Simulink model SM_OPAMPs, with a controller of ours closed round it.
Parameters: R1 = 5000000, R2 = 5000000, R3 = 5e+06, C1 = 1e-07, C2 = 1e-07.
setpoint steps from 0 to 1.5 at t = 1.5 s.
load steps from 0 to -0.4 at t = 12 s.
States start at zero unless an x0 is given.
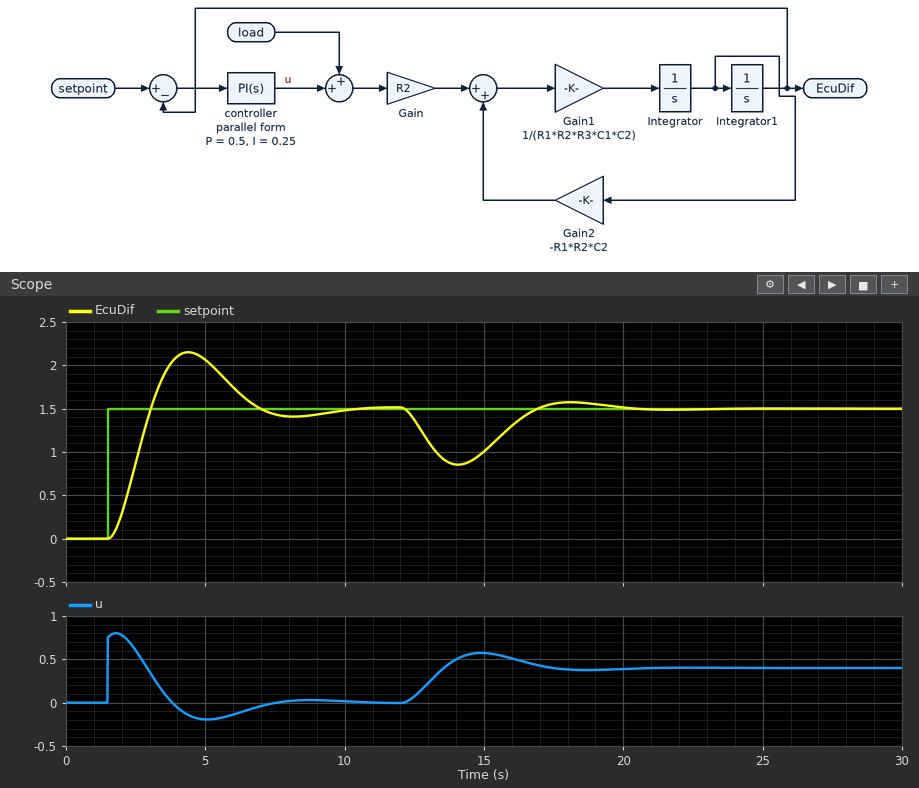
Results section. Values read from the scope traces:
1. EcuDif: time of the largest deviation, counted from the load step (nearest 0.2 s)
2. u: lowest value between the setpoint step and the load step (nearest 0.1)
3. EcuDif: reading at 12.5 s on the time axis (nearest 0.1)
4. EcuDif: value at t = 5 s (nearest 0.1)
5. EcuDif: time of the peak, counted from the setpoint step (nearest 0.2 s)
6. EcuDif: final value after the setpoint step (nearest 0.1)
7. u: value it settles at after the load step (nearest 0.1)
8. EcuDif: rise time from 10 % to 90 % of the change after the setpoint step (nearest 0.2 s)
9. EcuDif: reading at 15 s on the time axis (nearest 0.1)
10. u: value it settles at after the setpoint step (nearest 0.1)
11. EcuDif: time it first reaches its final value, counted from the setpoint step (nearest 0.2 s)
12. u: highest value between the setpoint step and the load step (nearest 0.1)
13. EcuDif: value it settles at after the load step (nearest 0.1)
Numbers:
2.0 s
-0.2
1.4
2.1
2.8 s
1.5
0.4
1.0 s
1.0
0.0
1.6 s
0.8
1.5
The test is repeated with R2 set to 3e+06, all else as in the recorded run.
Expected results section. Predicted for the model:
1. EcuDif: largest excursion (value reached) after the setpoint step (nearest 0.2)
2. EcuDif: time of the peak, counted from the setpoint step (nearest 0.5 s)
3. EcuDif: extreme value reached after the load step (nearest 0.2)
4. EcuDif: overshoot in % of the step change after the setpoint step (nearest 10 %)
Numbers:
2.2
3.0 s
0.8
40 %
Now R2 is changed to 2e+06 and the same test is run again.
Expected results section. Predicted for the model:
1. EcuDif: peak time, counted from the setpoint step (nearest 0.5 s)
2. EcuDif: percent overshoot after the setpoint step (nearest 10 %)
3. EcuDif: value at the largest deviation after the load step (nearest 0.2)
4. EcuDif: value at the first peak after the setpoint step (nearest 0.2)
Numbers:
3.0 s
40 %
0.8
2.2
